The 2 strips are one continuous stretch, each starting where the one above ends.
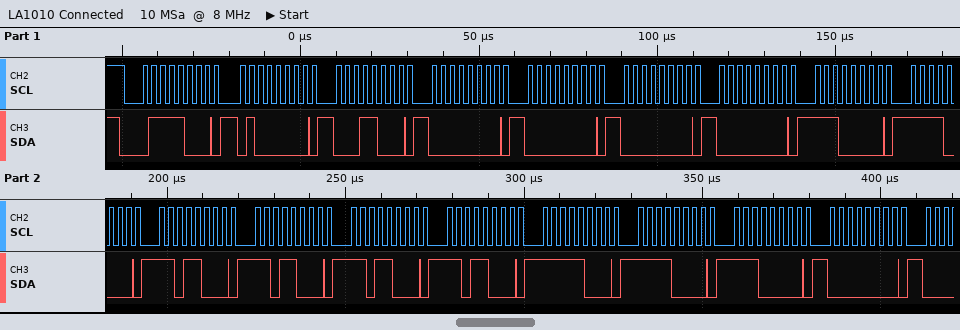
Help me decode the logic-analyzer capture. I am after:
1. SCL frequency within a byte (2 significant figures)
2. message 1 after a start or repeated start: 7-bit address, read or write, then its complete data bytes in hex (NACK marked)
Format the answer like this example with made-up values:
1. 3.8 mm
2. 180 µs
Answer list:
1. 400 kHz
2. 0x3C write: 40 18 00 00 00 00 E0 F0 D8 D8 D8 D8 F8 F0 E0 00
